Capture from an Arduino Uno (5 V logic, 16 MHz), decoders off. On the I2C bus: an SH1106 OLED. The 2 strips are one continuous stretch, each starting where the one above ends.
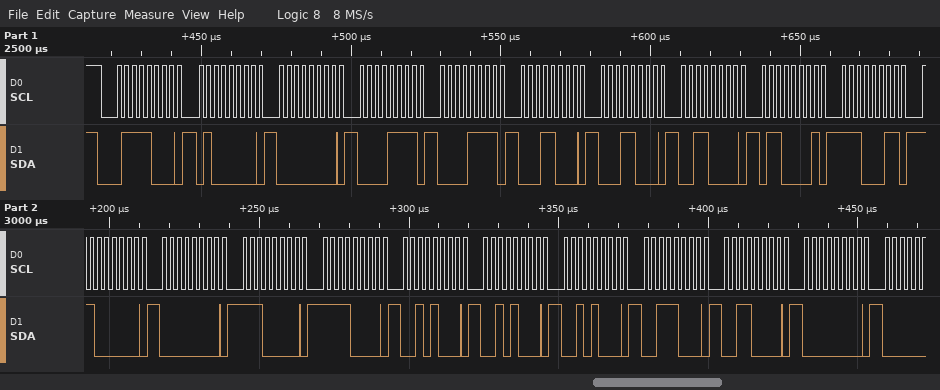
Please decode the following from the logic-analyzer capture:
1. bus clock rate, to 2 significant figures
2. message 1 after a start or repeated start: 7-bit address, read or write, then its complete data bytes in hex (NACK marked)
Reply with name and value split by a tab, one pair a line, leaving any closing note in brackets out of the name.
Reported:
bus clock rate, to 2 significant figures	400 kHz
message 1 after a start or repeated start: 7-bit address, read or write, then its complete data bytes in hex	0x3C write: 40 00 0F 0F 18 18 30 61 E3 C0 00 E0 F0 28 28 28 38 30 00
